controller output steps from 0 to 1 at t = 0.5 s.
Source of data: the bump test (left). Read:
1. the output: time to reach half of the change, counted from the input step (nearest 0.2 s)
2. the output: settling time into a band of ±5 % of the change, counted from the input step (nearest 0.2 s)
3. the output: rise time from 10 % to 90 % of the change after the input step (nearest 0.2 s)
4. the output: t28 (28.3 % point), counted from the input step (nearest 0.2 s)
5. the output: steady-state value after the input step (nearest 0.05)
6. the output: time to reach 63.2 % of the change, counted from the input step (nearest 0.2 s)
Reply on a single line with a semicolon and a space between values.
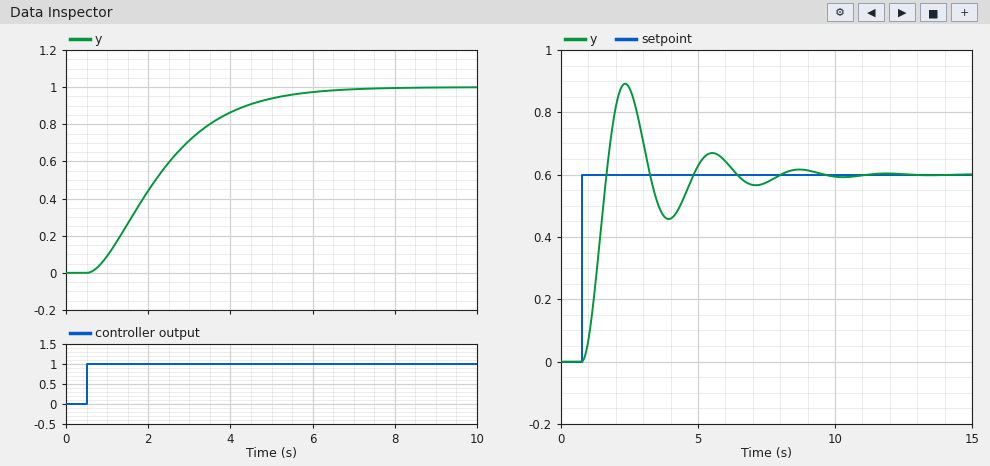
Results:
1.6 s; 4.8 s; 3.4 s; 1.0 s; 1.00; 2.2 s
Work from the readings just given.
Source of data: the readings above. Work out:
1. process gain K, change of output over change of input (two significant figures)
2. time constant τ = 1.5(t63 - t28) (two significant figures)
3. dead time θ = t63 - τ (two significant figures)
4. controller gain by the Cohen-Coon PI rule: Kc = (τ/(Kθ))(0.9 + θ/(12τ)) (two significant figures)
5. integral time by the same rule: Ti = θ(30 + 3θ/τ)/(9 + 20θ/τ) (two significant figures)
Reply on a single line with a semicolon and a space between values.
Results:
1.0; 1.8 s; 0.40 s; 4.1; 0.91 s
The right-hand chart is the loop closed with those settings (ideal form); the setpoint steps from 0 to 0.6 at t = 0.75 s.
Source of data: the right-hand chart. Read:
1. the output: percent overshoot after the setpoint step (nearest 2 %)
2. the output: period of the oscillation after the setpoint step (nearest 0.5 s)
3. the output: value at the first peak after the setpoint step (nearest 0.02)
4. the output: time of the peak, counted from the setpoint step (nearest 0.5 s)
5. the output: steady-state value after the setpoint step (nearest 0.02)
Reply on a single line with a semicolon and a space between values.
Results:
48 %; 3.0 s; 0.90; 1.5 s; 0.60
